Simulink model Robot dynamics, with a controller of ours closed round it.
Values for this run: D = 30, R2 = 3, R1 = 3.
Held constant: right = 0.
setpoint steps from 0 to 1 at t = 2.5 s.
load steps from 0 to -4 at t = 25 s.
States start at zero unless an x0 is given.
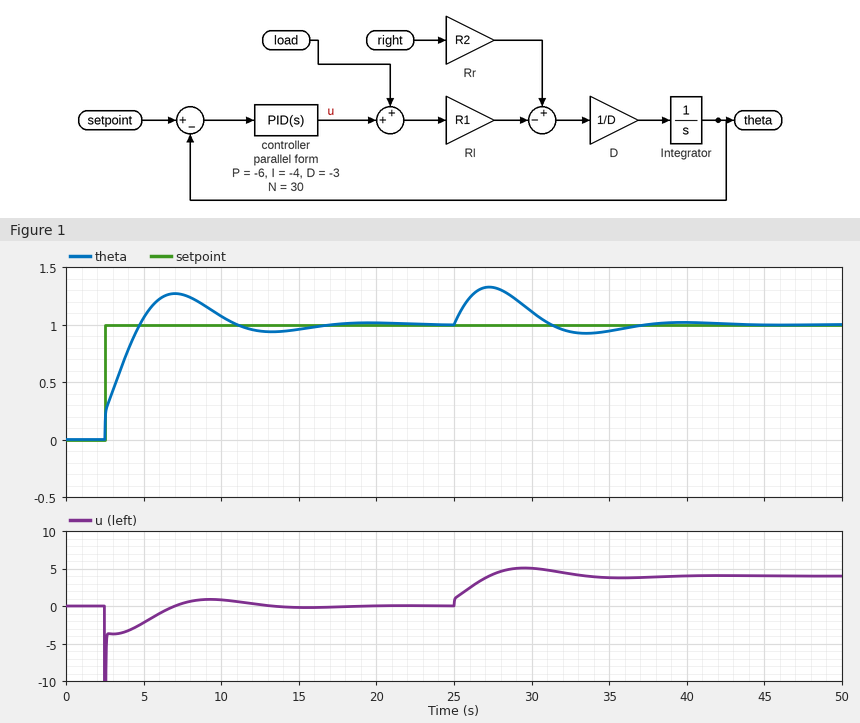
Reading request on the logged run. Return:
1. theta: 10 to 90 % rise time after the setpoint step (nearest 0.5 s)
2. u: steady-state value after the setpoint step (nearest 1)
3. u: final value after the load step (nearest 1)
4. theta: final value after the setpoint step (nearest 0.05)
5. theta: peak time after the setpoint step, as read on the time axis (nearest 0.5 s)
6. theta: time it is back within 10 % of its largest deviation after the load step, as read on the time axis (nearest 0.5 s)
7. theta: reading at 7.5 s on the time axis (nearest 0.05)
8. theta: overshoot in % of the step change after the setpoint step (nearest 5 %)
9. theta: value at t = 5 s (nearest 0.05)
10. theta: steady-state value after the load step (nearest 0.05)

2.0 s
0
4
1.00
7.0 s
36.0 s
1.25
25 %
1.05
1.00
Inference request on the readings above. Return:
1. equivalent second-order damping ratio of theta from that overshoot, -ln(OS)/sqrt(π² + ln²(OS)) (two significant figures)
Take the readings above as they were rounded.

0.40
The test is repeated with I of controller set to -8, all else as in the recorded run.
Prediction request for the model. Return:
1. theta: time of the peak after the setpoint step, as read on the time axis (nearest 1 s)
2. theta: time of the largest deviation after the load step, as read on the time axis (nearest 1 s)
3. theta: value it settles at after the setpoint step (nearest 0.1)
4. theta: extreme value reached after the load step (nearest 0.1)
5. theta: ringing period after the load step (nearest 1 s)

6 s
27 s
1.0
1.3
8 s
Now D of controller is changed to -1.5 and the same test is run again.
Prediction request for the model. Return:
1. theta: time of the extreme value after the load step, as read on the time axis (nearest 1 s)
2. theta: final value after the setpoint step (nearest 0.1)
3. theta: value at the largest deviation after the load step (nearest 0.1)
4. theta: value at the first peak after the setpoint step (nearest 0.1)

27 s
1.0
1.3
1.3
